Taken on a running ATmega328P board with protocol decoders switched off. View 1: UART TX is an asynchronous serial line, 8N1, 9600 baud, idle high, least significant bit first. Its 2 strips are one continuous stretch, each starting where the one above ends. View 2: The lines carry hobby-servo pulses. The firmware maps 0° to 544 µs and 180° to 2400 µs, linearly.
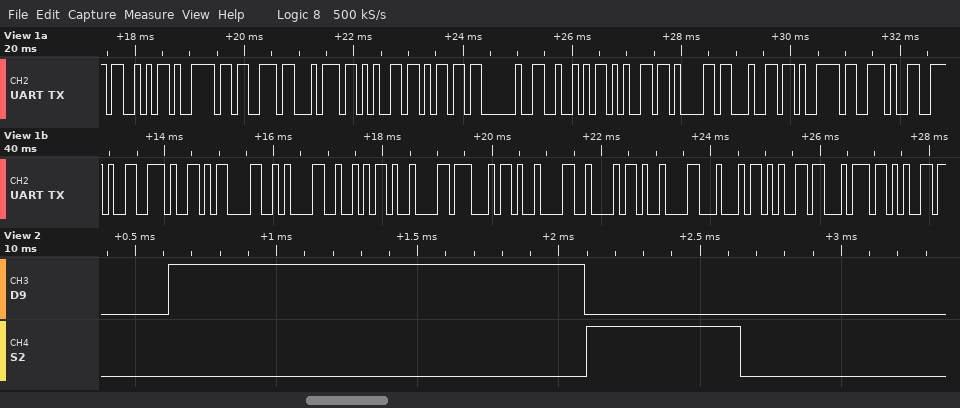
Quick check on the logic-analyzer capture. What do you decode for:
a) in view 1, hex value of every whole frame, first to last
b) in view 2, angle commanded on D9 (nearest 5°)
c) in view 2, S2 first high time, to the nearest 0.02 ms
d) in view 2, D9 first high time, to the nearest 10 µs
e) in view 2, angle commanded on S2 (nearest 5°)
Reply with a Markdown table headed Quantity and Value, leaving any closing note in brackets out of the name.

| Quantity | Value |
|---|---|
| in view 1, hex value of every whole frame, first to last | 0x53 0x79 0x73 0x74 0x65 0x6D 0x20 0x52 0x65 0x61 0x64 0x79 0x2E 0x2E 0x2E 0x0D 0x0A 0x52 0x09 0x47 0x09 0x42 0x09 0x44 0x65 0x74 0x65 |
| in view 2, angle commanded on D9 | 90° |
| in view 2, S2 first high time, to the nearest 0.02 ms | 0.54 ms |
| in view 2, D9 first high time, to the nearest 10 µs | 1470 µs |
| in view 2, angle commanded on S2 | 0° |
